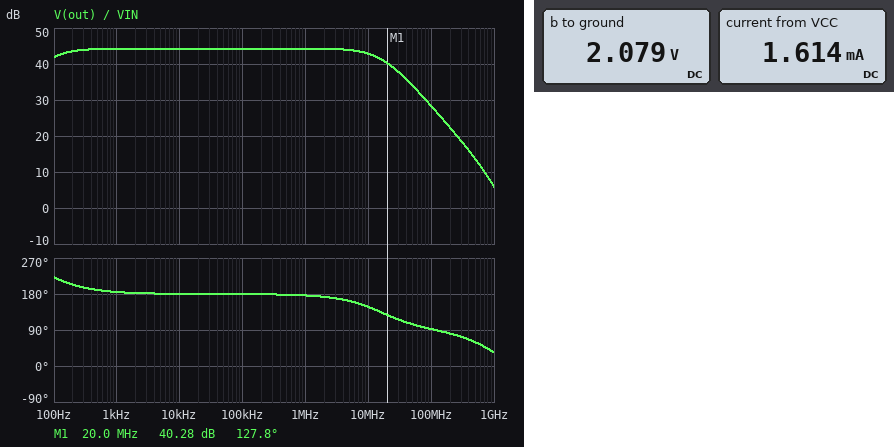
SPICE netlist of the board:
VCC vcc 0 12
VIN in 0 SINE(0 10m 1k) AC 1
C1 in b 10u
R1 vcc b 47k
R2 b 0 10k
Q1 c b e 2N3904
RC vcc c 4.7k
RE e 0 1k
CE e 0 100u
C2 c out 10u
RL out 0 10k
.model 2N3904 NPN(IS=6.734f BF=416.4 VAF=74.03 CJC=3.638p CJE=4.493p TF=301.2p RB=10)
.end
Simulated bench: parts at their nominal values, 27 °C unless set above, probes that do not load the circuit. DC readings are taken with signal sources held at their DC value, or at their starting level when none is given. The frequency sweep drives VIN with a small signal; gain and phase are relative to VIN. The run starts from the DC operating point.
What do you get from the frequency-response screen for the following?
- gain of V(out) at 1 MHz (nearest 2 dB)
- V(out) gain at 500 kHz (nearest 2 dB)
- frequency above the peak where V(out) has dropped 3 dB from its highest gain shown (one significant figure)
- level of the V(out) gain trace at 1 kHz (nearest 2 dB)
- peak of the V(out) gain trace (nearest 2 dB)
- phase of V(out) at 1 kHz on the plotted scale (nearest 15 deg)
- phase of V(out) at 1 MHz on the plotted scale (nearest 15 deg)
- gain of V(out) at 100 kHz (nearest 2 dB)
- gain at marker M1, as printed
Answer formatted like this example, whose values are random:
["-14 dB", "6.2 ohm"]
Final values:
["44 dB", "44 dB", "20 MHz", "44 dB", "44 dB", "180 deg", "180 deg", "44 dB", "40.28 dB"]
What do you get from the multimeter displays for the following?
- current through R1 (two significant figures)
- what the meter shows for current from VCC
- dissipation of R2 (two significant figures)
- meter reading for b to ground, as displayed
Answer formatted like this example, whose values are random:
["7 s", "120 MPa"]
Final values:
["210 µA", "1.614 mA", "430 µW", "2.079 V"]
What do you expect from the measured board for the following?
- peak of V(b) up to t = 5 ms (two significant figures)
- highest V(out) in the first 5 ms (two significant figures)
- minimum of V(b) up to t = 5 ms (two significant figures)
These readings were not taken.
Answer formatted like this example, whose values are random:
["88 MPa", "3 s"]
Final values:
["2.1 V", "1.5 V", "2.1 V"]
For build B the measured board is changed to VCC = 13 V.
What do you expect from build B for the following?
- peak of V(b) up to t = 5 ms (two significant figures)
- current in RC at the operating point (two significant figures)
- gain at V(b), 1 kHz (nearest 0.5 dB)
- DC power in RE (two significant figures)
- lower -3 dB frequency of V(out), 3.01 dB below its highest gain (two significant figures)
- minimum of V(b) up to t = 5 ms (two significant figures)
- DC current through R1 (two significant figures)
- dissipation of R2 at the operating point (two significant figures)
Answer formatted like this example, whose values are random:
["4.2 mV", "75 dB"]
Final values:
["2.3 V", "1.6 mA", "0 dB", "2.5 mW", "95 Hz", "2.2 V", "230 µA", "510 µW"]
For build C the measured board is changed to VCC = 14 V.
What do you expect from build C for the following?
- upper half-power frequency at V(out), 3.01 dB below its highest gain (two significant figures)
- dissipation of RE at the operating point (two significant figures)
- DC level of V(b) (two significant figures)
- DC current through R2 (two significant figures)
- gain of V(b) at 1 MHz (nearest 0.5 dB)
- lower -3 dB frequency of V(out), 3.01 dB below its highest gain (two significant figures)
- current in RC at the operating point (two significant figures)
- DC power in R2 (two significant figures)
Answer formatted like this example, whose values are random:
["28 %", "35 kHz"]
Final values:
["15 MHz", "3.0 mW", "2.4 V", "240 µA", "0 dB", "100 Hz", "1.7 mA", "590 µW"]
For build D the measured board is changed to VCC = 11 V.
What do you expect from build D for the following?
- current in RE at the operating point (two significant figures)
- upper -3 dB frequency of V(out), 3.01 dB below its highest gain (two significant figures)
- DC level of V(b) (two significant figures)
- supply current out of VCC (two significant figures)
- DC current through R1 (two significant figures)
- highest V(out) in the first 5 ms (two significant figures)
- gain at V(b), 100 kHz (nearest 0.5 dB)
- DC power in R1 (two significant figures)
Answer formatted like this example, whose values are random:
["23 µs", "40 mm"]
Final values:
["1.2 mA", "17 MHz", "1.9 V", "1.4 mA", "190 µA", "1.3 V", "0 dB", "1.8 mW"]
